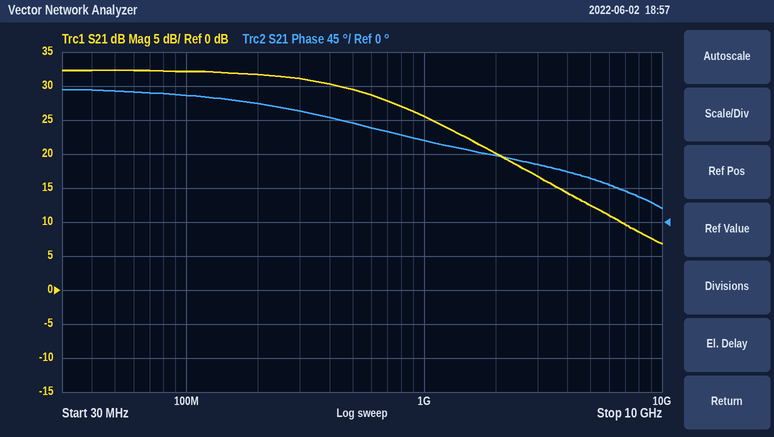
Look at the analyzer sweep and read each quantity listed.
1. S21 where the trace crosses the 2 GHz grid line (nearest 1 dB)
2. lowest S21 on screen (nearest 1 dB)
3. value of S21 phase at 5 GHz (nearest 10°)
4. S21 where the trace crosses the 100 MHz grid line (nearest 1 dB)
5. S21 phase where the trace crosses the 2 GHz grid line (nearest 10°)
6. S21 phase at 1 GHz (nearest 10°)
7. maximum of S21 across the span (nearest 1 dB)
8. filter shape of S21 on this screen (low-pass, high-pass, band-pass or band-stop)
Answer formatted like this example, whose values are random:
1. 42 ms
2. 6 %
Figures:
1. 20 dB
2. 7 dB
3. 60°
4. 32 dB
5. 90°
6. 110°
7. 32 dB
8. low-pass
